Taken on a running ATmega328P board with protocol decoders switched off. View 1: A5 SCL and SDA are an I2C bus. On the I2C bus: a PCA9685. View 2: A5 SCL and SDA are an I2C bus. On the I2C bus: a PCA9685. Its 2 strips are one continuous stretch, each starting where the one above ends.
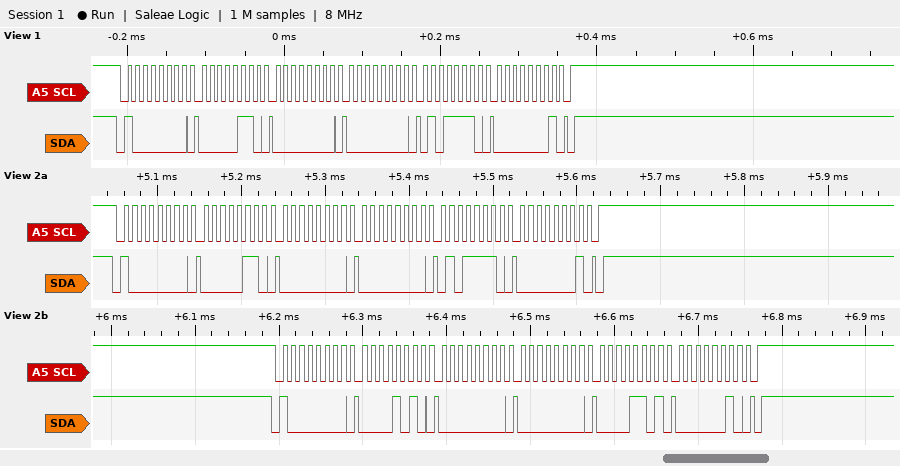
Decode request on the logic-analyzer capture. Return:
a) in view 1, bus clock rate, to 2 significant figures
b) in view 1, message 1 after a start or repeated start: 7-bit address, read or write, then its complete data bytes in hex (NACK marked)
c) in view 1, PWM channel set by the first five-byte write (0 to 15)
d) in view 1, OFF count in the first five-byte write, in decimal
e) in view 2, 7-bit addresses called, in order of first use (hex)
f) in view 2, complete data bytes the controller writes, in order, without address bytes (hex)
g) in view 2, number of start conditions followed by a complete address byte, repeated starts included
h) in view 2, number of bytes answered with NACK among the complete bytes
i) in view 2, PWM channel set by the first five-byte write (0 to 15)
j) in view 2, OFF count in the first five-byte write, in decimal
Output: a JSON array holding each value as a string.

["100 kHz", "0x40 write: 06 00 00 5E 01", "0", "350", "0x40", "06 00 00 5E 01 0A 00 00 0D 02", "2", "0", "0", "350"]
